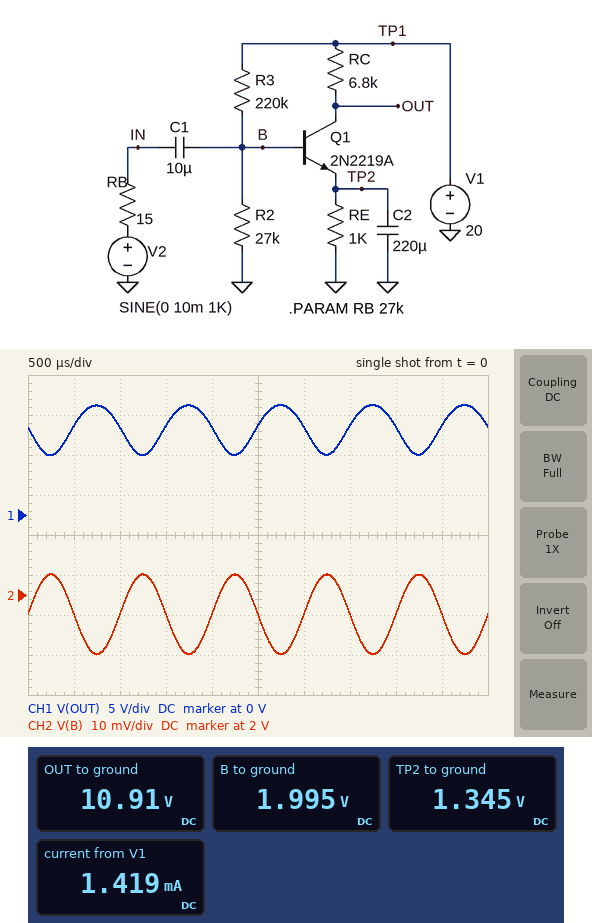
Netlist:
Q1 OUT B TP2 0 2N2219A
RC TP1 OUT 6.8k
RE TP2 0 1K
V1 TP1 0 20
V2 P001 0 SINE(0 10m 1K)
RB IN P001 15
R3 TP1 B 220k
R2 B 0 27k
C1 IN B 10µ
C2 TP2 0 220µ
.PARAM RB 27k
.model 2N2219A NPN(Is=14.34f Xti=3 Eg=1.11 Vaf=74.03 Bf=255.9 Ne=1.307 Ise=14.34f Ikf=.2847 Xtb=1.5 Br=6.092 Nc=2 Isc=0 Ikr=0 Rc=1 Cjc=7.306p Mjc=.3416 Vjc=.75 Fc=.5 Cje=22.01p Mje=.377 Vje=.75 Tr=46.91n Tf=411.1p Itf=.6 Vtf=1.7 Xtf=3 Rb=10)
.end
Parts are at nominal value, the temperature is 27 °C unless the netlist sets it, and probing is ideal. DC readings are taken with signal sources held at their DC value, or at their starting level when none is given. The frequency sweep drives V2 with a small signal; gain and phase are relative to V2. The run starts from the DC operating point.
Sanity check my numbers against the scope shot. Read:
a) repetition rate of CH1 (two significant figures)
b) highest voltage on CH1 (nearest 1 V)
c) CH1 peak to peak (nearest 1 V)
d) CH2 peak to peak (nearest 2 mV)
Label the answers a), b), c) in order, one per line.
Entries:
a) 1.0 kHz
b) 14 V
c) 6 V
d) 20 mV
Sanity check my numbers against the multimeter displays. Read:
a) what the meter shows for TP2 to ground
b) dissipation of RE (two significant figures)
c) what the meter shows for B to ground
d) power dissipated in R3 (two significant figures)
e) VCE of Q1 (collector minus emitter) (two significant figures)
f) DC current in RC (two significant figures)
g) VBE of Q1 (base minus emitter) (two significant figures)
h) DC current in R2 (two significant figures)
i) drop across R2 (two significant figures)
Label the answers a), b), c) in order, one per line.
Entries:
a) 1.345 V
b) 1.8 mW
c) 1.995 V
d) 1.5 mW
e) 9.6 V
f) 1.3 mA
g) 650 mV
h) 74 µA
i) 2.0 V
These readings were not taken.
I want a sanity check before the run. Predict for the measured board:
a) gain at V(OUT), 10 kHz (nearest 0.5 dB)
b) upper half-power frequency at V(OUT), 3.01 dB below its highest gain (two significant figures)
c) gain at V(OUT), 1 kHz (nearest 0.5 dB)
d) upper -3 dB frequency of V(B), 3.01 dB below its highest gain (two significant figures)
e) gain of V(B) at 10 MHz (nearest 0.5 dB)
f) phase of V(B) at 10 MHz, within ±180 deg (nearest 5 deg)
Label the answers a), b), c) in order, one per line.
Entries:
a) 50.0 dB
b) 3.7 MHz
c) 50.0 dB
d) 9.8 MHz
e) -3.0 dB
f) -10 deg
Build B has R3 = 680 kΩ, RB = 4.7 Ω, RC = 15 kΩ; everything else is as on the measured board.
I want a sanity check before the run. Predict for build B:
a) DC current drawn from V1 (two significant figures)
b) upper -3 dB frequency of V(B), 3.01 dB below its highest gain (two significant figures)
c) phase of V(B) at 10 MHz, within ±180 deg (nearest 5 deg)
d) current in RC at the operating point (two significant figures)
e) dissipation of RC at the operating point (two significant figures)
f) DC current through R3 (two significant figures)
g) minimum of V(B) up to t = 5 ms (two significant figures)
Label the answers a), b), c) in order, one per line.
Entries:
a) 170 µA
b) 1.1 GHz
c) 0 deg
d) 150 µA
e) 320 µW
f) 28 µA
g) 730 mV
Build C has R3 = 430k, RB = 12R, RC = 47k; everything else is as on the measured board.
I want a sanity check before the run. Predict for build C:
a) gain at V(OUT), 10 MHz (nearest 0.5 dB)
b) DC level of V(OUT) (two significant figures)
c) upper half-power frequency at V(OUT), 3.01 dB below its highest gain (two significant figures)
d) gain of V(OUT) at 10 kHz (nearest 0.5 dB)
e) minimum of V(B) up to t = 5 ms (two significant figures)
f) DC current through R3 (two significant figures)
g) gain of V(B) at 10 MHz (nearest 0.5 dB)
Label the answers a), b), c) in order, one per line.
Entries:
a) 14.5 dB
b) 510 mV
c) 2.2 MHz
d) 27.5 dB
e) 1.0 V
f) 44 µA
g) -1.5 dB
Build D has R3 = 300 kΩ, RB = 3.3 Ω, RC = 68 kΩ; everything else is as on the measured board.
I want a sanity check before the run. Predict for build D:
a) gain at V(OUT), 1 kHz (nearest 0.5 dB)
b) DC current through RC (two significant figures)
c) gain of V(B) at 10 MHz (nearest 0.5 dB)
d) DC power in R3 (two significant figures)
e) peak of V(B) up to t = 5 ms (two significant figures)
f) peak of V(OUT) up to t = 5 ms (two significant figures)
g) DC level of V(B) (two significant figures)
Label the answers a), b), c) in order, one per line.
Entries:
a) 4.0 dB
b) 290 µA
c) -0.5 dB
d) 1.2 mW
e) 950 mV
f) 390 mV
g) 940 mV
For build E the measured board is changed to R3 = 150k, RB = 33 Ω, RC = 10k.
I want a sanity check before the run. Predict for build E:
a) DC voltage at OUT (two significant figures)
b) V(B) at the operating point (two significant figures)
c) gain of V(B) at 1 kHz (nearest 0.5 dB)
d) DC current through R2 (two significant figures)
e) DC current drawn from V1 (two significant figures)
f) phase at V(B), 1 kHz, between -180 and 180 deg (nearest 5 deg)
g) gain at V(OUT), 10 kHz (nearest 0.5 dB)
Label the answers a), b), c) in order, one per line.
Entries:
a) 1.9 V
b) 2.5 V
c) -2.5 dB
d) 92 µA
e) 1.9 mA
f) 5 deg
g) 23.0 dB
